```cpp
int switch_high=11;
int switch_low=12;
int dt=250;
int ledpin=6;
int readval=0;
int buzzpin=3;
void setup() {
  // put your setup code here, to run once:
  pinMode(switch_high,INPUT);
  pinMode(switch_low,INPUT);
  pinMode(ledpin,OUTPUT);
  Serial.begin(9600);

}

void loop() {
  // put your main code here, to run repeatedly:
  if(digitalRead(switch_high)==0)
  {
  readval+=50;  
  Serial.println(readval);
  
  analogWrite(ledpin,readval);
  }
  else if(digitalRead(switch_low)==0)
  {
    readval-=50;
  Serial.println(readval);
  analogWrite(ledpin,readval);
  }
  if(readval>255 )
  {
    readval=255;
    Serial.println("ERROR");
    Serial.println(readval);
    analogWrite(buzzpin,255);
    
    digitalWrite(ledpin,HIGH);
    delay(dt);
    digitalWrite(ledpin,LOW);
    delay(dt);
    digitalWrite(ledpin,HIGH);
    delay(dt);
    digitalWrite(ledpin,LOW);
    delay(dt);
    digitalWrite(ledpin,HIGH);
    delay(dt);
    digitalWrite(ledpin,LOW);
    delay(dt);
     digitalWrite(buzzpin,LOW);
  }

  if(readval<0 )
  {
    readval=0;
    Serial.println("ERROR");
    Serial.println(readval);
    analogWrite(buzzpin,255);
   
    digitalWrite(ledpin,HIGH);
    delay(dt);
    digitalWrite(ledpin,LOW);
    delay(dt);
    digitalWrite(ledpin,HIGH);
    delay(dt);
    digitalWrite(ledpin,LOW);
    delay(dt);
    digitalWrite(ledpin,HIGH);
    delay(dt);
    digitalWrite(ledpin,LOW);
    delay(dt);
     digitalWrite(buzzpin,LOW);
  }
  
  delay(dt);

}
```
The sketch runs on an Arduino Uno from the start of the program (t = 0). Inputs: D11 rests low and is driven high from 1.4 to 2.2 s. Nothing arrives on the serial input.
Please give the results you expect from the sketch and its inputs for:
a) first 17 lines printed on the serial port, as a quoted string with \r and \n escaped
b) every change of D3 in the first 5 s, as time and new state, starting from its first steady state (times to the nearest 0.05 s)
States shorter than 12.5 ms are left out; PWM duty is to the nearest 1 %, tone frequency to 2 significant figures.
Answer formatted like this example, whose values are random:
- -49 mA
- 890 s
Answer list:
- "50\r\n100\r\n150\r\n200\r\n250\r\n300\r\nERROR\r\n255\r\n305\r\nERROR\r\n255\r\n305\r\nERROR\r\n255\r\n305\r\nERROR\r\n255\r\n"
- 1.25 s high; 2.75 s low; 3 s high; 4.5 s low; 4.75 s high
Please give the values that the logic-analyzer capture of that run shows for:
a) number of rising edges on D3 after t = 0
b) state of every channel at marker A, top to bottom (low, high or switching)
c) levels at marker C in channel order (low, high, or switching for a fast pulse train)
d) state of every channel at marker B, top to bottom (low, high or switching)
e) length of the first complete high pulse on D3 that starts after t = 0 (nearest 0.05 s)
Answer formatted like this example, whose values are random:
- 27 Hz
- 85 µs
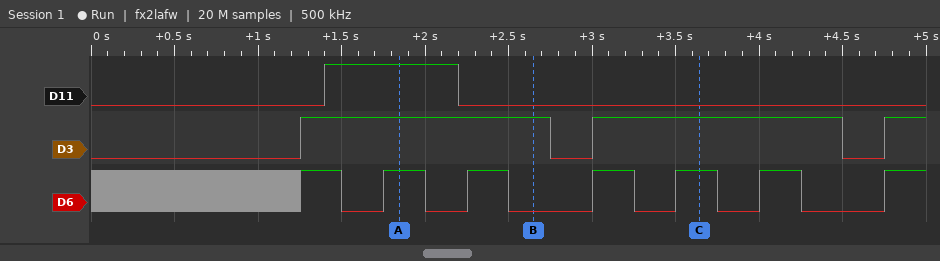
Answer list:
- 3
- D11 high, D3 high, D6 high
- D11 low, D3 high, D6 high
- D11 low, D3 high, D6 low
- 1.50 s
